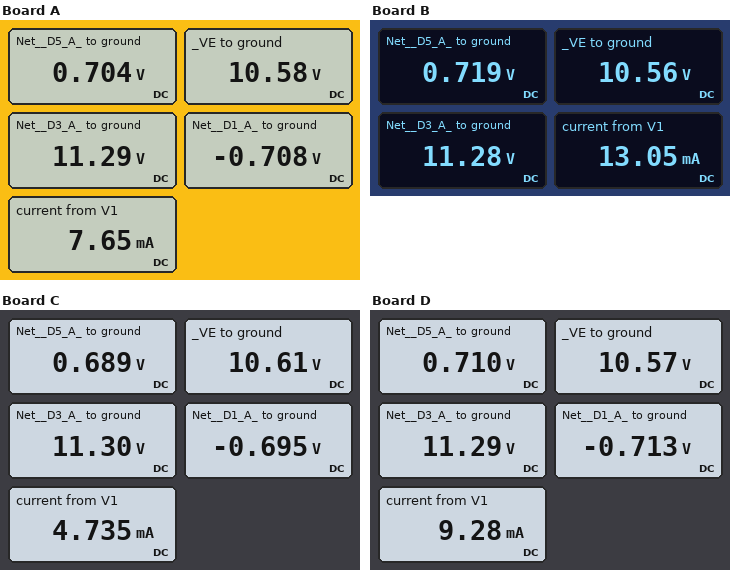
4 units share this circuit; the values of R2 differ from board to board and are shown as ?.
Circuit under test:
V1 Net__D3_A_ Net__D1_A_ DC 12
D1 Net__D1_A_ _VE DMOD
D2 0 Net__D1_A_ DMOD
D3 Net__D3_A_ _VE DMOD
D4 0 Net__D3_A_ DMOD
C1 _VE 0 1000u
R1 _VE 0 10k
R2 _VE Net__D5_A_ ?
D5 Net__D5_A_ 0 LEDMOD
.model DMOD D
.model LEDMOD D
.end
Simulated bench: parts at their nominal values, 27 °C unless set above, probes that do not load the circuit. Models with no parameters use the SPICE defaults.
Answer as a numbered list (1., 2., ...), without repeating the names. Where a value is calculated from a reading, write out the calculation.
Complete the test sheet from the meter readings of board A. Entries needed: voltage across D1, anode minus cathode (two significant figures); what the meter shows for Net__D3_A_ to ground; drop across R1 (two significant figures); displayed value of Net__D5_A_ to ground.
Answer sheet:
1. -708 mV - 10.58 V = -11 V
2. 11.29 V
3. 10.58 V = 11 V
4. 0.704 V
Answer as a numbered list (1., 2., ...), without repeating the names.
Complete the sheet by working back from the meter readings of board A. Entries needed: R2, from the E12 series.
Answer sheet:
1. 1.5 kΩ
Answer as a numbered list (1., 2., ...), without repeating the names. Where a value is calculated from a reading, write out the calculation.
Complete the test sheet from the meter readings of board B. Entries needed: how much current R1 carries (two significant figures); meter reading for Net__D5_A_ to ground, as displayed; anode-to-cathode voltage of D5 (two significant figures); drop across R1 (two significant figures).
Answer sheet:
1. (10.56 V) / 10 kΩ = 1.1 mA
2. 0.719 V
3. 719 mV = 720 mV
4. 10.56 V = 11 V
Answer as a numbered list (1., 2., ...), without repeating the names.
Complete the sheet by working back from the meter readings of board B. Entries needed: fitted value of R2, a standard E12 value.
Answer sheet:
1. 820 Ω
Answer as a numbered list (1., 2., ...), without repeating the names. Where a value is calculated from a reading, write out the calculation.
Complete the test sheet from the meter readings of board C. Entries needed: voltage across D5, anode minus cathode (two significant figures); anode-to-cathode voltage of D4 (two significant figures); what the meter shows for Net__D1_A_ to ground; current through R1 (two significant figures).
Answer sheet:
1. 689 mV = 690 mV
2. 0 V - 11.3 V = -11 V
3. -0.695 V
4. (10.61 V) / 10 kΩ = 1.1 mA
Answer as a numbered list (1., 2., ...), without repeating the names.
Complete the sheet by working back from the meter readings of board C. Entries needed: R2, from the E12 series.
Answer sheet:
1. 2.7 kΩ
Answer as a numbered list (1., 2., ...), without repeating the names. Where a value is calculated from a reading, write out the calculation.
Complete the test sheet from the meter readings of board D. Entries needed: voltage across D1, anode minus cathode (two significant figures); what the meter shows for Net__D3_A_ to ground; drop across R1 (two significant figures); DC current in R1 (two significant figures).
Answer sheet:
1. -713 mV - 10.57 V = -11 V
2. 11.29 V
3. 10.57 V = 11 V
4. (10.57 V) / 10 kΩ = 1.1 mA
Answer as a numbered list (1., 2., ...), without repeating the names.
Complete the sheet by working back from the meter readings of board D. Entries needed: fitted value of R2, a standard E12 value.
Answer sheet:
1. 1.2 kΩ
